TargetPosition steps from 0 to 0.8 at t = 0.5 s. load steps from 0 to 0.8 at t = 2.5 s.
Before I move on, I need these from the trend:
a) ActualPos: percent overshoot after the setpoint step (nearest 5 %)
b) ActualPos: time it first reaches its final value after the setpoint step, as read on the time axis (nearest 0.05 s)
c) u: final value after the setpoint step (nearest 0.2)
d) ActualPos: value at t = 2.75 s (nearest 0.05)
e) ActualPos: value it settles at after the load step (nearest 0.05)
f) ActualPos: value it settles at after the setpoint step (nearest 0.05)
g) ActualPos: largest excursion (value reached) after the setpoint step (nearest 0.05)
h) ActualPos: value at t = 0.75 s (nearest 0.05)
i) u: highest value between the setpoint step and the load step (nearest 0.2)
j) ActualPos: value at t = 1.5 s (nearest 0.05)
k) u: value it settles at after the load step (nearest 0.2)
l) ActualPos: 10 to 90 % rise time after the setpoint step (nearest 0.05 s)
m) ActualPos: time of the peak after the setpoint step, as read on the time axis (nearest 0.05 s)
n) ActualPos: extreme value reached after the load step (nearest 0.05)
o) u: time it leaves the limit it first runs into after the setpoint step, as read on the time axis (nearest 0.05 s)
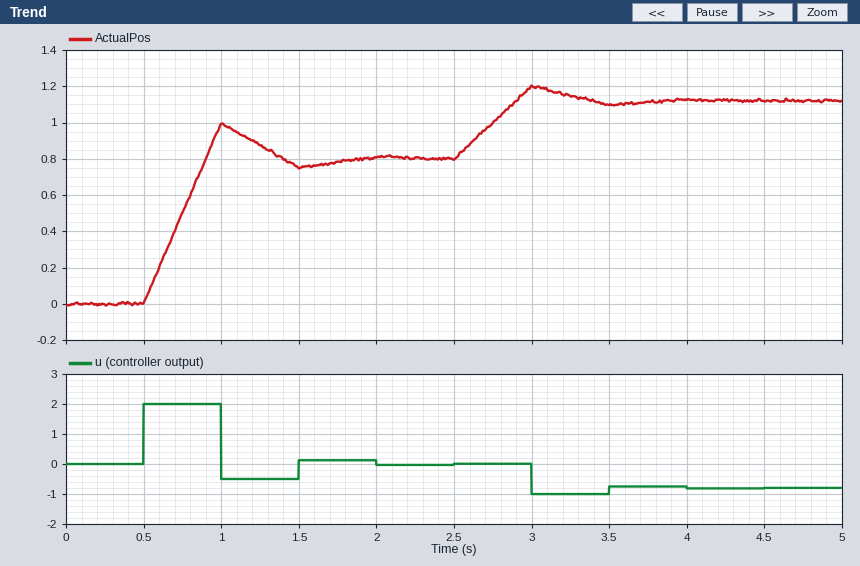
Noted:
25 %
0.90 s
0.0
1.00
1.10
0.80
1.00
0.50
2.0
0.75
-0.8
0.30 s
1.00 s
1.20
1.00 s
